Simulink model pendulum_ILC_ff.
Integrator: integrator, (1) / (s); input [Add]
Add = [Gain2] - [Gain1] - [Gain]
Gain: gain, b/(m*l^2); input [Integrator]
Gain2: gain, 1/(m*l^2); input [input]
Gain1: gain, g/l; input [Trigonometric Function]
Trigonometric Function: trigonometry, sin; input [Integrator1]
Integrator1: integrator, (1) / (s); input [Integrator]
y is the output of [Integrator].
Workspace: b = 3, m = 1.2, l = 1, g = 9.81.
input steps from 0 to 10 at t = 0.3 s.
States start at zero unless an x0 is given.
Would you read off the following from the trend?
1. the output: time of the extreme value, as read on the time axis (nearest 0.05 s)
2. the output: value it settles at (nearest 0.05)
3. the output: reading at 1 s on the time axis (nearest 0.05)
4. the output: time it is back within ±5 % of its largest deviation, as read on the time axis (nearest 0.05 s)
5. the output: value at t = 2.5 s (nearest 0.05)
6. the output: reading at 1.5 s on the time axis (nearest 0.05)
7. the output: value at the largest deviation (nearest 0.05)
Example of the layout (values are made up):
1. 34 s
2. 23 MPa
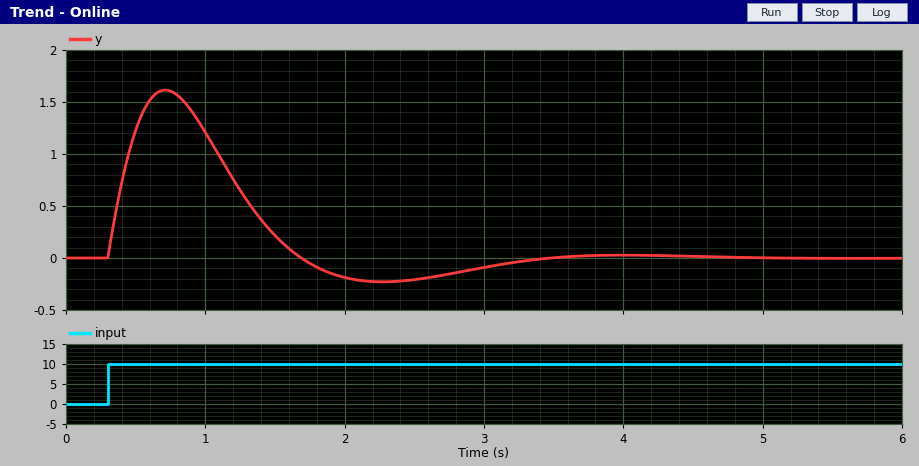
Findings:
1. 0.70 s
2. 0.00
3. 1.20
4. 3.05 s
5. -0.20
6. 0.20
7. 1.60
